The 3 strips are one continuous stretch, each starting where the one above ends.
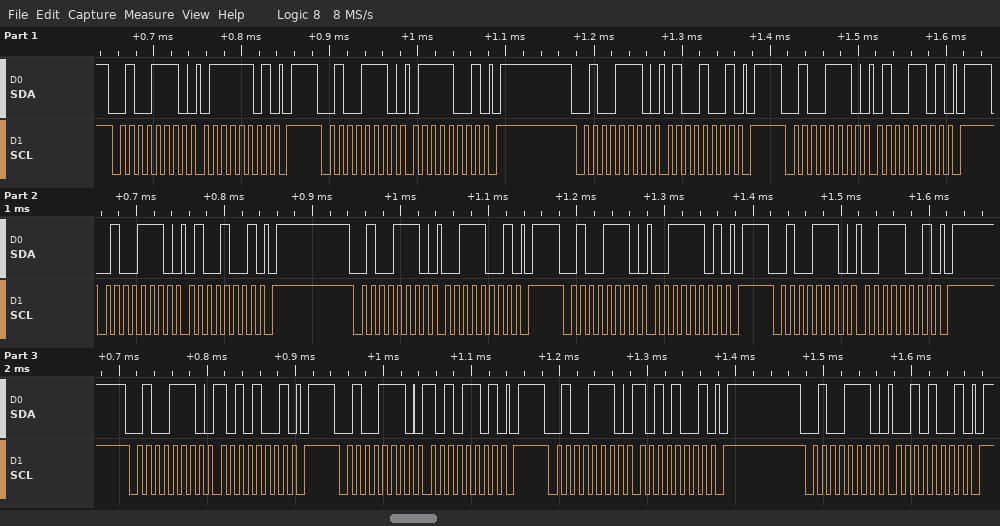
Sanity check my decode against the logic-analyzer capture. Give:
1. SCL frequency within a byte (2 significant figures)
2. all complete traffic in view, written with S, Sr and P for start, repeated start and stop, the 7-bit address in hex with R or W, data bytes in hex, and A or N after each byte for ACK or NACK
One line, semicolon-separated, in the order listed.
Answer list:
100 kHz; S 27W A 7D A P S 27W A 79 A P S 27W A 49 A P S 27W A 4D A P S 27W A 49 A P S 27W A 39 A P S 27W A 3D A P S 27W A 39 A P S 27W A A9 A P S 27W A AD A P S 27W A A9 A P S 27W A 29 A P
